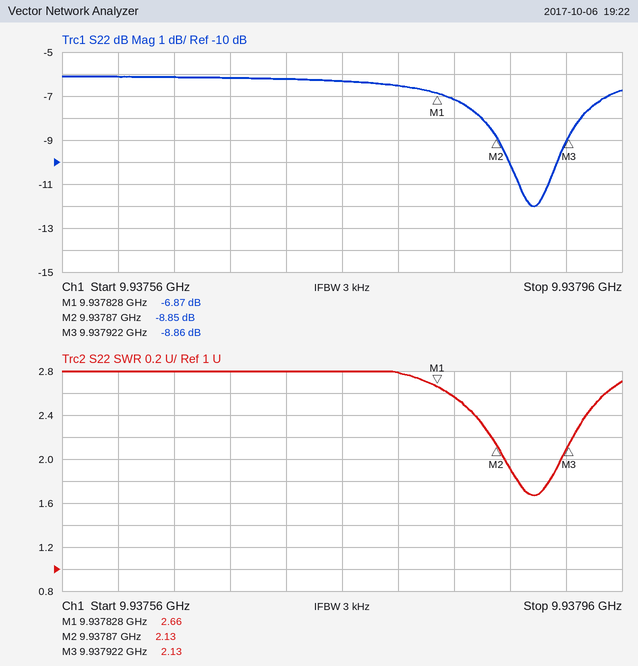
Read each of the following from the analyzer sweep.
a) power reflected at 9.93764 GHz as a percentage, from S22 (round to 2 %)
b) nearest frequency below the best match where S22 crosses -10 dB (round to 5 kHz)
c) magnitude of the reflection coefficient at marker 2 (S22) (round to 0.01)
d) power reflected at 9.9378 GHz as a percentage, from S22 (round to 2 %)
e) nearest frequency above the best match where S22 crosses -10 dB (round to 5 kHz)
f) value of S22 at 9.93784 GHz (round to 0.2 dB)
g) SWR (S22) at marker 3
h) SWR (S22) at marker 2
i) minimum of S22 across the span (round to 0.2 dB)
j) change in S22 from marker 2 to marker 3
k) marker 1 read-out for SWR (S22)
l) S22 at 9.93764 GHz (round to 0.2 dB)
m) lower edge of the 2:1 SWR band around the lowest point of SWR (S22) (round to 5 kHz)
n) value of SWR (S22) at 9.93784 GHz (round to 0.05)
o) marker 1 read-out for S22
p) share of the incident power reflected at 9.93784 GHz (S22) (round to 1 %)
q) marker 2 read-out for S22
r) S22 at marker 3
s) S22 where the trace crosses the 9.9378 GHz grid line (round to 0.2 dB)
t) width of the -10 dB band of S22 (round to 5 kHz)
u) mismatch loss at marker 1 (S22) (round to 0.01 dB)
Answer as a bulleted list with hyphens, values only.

- 24 %
- 9.937880 GHz
- 0.36
- 22 %
- 9.937915 GHz
- -7.2 dB
- 2.13
- 2.13
- -12.0 dB
- -0.01 dB
- 2.66
- -6.2 dB
- 9.937875 GHz
- 2.55
- -6.87 dB
- 19 %
- -8.85 dB
- -8.86 dB
- -6.6 dB
- 35 kHz
- 1.00 dB
